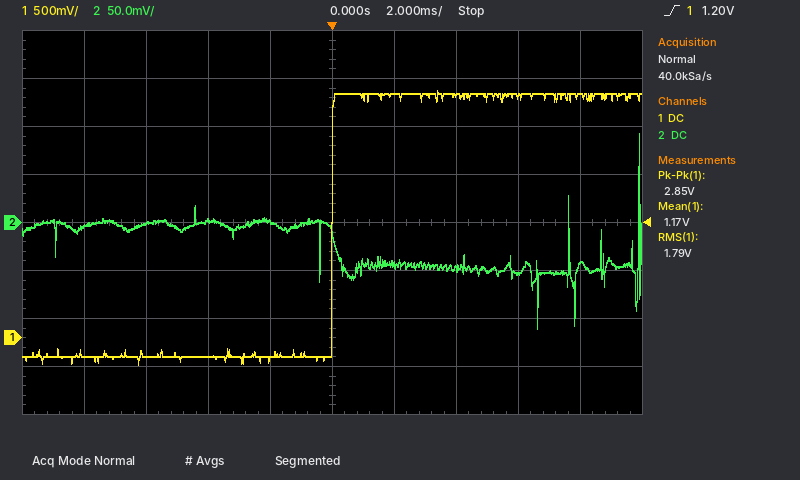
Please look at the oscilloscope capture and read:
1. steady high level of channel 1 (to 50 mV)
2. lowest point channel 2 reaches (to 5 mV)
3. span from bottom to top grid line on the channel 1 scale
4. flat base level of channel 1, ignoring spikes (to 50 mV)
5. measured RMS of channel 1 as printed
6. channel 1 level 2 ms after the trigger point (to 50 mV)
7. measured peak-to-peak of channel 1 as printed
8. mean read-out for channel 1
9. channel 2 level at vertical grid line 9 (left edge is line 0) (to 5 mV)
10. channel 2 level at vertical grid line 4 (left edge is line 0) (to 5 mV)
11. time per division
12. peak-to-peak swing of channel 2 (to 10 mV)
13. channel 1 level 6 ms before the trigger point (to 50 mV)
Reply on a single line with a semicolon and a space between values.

2.55 V; -110 mV; 4 V; -200 mV; 1.79 V; 2.55 V; 2.85 V; 1.17 V; -45 mV; 0 mV; 2 ms; 200 mV; -200 mV
